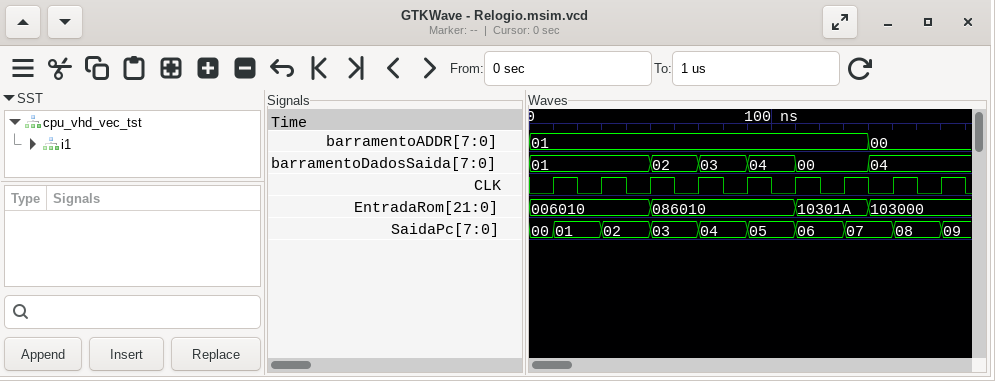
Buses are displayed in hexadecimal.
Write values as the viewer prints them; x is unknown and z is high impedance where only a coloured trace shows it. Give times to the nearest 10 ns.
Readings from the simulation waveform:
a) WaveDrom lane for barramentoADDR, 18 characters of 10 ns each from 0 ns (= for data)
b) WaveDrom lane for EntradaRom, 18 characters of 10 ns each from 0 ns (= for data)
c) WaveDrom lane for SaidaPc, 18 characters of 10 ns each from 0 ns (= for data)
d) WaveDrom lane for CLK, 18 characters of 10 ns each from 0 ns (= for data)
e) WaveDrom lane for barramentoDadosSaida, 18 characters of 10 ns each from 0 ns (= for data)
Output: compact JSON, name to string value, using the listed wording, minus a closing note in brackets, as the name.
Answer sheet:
{"WaveDrom lane for barramentoADDR, 18 characters of 10 ns each from 0 ns": "{name: 'barramentoADDR', wave: '=.............=...', data: '01 00'}", "WaveDrom lane for EntradaRom, 18 characters of 10 ns each from 0 ns": "{name: 'EntradaRom', wave: '=....=.....=..=...', data: '006010 086010 10301A 103000'}", "WaveDrom lane for SaidaPc, 18 characters of 10 ns each from 0 ns": "{name: 'SaidaPc', wave: '==.=.=.=.=.=.=.=.=', data: '00 01 02 03 04 05 06 07 08 09'}", "WaveDrom lane for CLK, 18 characters of 10 ns each from 0 ns": "{name: 'CLK', wave: '010101010101010101'}", "WaveDrom lane for barramentoDadosSaida, 18 characters of 10 ns each from 0 ns": "{name: 'barramentoDadosSaida', wave: '=....=.=.=.=..=...', data: '01 02 03 04 00 04'}"}
